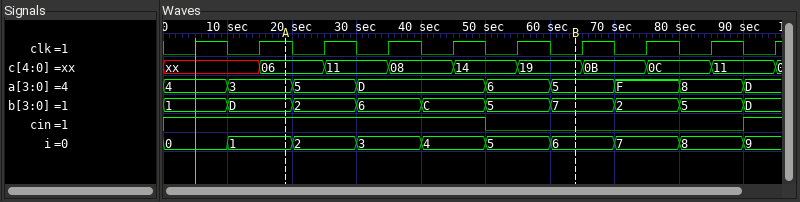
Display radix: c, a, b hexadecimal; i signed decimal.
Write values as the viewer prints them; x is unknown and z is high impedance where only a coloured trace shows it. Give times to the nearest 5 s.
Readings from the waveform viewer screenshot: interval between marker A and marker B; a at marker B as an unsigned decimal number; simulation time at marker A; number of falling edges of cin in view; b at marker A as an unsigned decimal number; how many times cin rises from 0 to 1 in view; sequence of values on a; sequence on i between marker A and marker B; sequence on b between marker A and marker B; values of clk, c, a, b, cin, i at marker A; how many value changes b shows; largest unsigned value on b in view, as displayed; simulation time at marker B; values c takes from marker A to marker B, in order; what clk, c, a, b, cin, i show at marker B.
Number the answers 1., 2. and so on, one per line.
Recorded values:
1. 45 s
2. 5
3. 20 s
4. 1
5. 13
6. 1
7. 4, 3, 5, D, 6, 5, F, 8, D
8. 1, 2, 3, 4, 5, 6
9. D, 2, 6, C, 5, 7
10. clk=1, c=06, a=3, b=D, cin=1, i=1
11. 9
12. D
13. 65 s
14. 06, 11, 08, 14, 19
15. clk=0, c=19, a=5, b=7, cin=0, i=6
